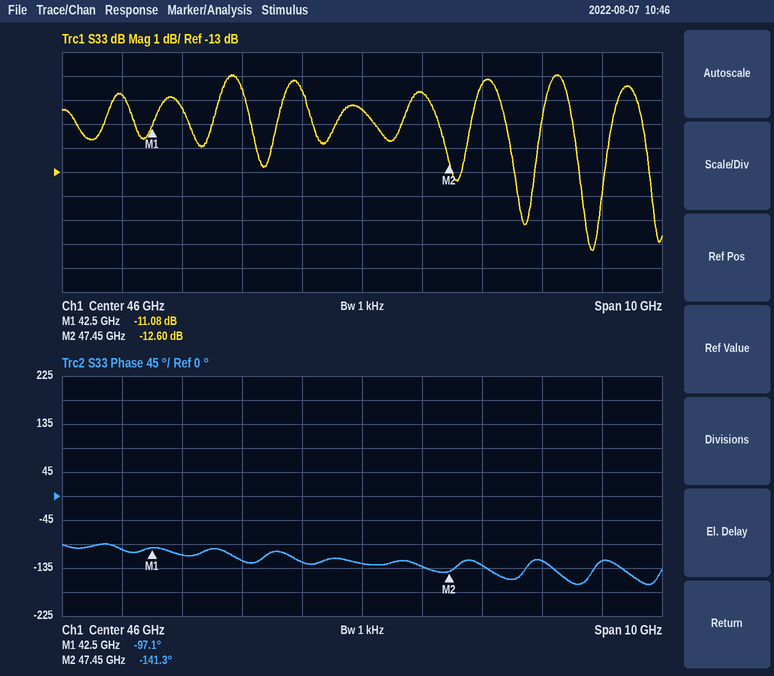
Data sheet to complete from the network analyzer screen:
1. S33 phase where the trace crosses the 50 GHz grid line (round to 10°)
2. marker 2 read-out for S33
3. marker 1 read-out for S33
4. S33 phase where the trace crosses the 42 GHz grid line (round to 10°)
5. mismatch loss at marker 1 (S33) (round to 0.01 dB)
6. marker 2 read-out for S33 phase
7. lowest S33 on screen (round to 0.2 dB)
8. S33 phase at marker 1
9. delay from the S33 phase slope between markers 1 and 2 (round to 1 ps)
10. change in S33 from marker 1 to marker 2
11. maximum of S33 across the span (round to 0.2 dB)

-120°
-12.60 dB
-11.08 dB
-100°
0.35 dB
-141.3°
-16.2 dB
-97.1°
25 ps
-1.52 dB
-9.0 dB
